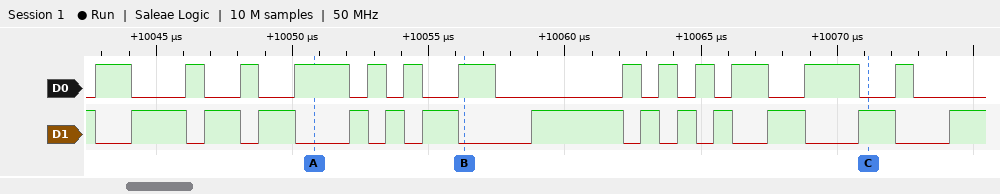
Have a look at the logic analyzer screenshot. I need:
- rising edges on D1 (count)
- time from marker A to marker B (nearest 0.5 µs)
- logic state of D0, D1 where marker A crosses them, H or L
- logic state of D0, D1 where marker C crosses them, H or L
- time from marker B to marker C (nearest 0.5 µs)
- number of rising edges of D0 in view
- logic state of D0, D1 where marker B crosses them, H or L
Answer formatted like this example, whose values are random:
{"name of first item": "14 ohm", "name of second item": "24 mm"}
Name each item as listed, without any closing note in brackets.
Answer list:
{"rising edges on D1": "13", "time from marker A to marker B": "5.5 µs", "logic state of D0, D1 where marker A crosses them, H or L": "D0=H, D1=L", "logic state of D0, D1 where marker C crosses them, H or L": "D0=L, D1=H", "time from marker B to marker C": "15 µs", "number of rising edges of D0 in view": "13", "logic state of D0, D1 where marker B crosses them, H or L": "D0=H, D1=L"}
